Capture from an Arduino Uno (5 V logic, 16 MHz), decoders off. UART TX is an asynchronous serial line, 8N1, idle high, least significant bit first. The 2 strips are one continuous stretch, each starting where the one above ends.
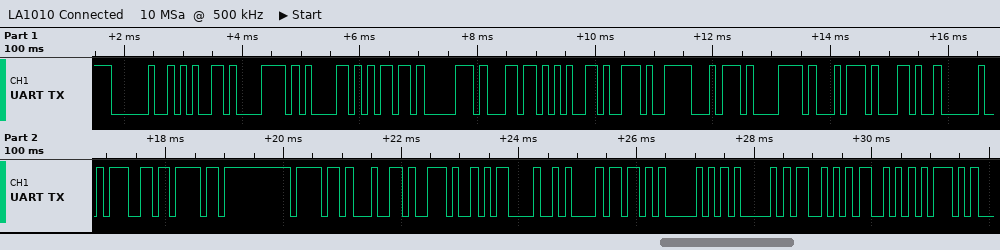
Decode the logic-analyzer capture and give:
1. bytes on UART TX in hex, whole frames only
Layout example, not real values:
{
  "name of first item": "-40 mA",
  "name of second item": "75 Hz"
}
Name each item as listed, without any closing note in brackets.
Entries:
{
  "bytes on UART TX in hex, whole frames only": "20 65 78 61 6D 70 6C 65 2E 74 78 74 2C 20 67 6F 6F 64 2E 0D 0A 5B 50 41 53 53 5D"
}
